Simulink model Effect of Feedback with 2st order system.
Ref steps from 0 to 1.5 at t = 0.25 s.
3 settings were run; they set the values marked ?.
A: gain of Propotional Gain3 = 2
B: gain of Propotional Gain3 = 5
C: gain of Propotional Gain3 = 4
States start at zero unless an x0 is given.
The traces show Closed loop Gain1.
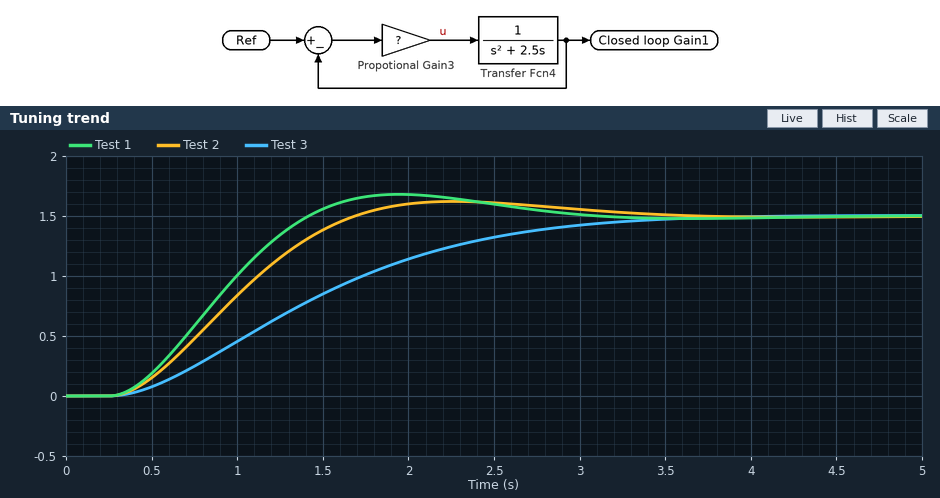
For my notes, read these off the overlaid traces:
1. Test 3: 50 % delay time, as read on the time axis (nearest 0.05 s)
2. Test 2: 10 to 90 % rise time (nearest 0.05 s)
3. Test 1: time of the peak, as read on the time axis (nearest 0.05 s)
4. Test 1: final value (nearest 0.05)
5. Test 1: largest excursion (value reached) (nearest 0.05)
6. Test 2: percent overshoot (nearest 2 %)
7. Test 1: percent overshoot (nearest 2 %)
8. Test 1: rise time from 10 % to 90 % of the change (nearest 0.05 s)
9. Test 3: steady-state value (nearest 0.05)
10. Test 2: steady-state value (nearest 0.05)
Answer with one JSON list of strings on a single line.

["1.35 s", "0.95 s", "1.95 s", "1.50", "1.70", "8 %", "12 %", "0.80 s", "1.50", "1.50"]
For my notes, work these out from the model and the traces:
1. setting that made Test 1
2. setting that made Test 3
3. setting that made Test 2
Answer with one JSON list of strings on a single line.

["B", "A", "C"]
